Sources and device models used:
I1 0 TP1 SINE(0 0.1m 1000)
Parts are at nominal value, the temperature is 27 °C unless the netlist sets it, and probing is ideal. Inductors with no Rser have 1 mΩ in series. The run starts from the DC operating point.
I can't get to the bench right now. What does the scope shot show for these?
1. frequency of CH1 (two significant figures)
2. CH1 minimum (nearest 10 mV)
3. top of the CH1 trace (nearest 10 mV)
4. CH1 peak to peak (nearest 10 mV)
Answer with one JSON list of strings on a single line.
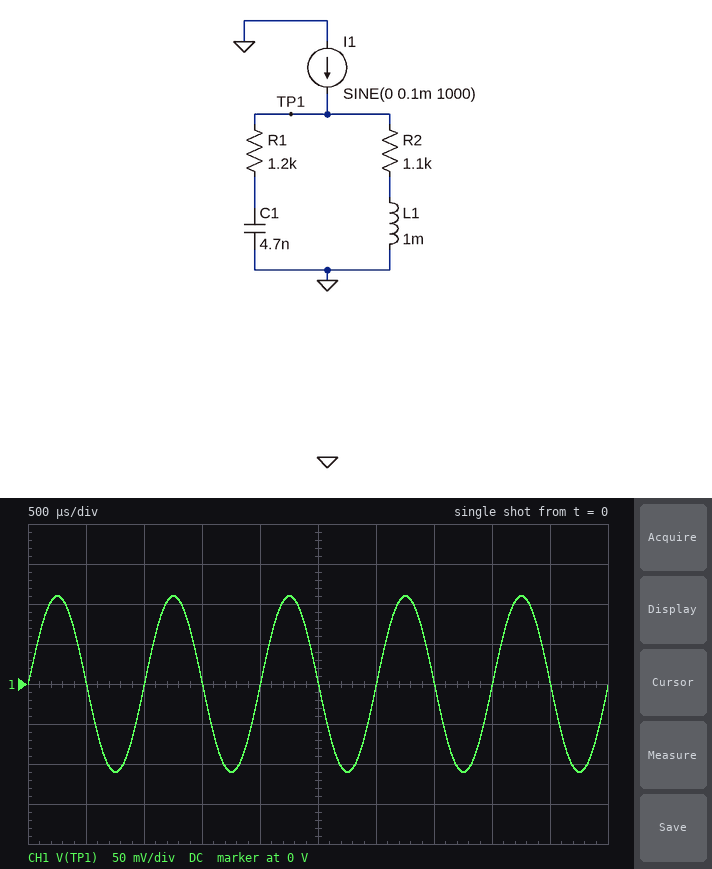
["1.0 kHz", "-110 mV", "110 mV", "220 mV"]
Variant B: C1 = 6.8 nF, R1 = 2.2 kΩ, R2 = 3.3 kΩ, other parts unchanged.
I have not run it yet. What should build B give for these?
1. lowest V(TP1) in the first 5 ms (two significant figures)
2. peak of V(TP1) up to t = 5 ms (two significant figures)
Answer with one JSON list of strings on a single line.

["-320 mV", "320 mV"]
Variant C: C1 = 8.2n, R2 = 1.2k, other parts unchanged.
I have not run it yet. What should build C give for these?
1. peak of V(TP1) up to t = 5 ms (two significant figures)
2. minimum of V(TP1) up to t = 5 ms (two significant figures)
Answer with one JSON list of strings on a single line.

["120 mV", "-120 mV"]
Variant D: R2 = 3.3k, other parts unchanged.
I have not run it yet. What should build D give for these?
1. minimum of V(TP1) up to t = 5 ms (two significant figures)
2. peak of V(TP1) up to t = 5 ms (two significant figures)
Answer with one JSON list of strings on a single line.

["-330 mV", "330 mV"]
